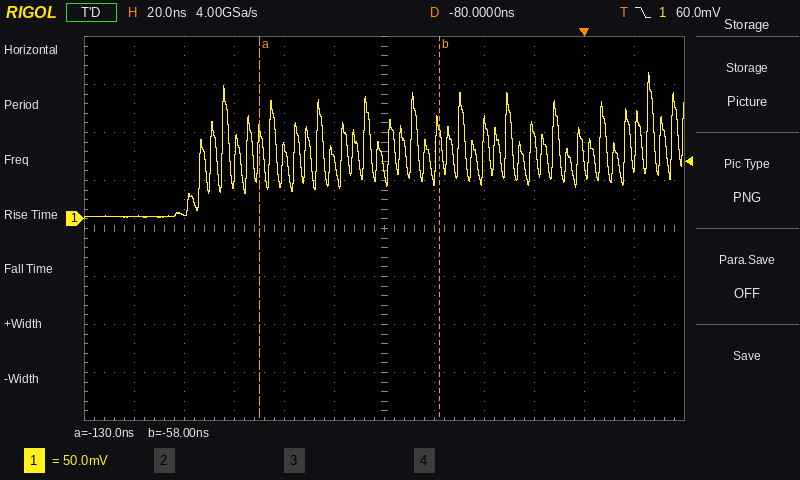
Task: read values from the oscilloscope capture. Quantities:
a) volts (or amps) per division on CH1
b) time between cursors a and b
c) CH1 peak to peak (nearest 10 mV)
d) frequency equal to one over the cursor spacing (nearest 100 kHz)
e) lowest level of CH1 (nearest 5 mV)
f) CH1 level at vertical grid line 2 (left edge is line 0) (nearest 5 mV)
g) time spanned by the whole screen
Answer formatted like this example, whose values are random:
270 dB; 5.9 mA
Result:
50 mV; 72 ns; 150 mV; 13.9 MHz; 0 mV; 5 mV; 240 ns
